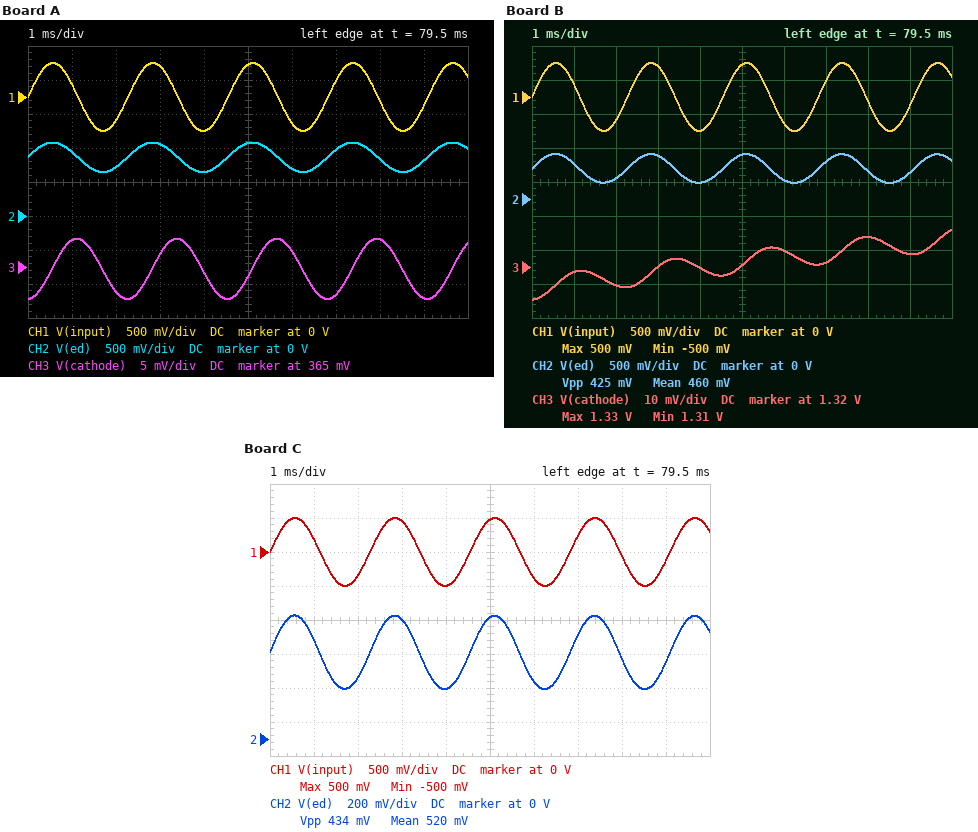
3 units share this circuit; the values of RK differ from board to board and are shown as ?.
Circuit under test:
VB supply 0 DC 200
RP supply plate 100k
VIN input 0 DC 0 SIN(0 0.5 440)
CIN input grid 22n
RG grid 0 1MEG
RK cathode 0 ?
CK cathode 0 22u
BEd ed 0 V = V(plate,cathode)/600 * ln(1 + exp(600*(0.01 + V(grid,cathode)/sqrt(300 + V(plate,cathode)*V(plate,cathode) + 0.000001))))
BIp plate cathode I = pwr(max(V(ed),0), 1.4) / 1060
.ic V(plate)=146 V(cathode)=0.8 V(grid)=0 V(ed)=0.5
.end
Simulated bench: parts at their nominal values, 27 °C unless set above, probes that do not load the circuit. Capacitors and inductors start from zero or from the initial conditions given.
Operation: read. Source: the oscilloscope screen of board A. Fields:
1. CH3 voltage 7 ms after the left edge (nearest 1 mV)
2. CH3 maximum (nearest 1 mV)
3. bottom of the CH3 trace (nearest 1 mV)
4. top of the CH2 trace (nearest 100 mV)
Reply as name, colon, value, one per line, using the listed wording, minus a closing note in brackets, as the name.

CH3 voltage 7 ms after the left edge: 361 mV
CH3 maximum: 369 mV
bottom of the CH3 trace: 360 mV
top of the CH2 trace: 1.1 V
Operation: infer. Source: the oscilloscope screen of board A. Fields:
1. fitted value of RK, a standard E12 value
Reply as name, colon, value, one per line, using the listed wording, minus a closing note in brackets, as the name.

fitted value of RK, a standard E12 value: 470 Ω
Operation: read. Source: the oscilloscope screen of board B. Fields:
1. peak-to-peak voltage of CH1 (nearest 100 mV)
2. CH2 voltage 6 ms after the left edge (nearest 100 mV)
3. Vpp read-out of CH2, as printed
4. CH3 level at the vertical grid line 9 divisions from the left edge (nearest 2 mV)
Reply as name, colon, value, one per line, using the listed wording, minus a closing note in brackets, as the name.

peak-to-peak voltage of CH1: 1.0 V
CH2 voltage 6 ms after the left edge: 300 mV
Vpp read-out of CH2, as printed: 425 mV
CH3 level at the vertical grid line 9 divisions from the left edge: 1.324 V
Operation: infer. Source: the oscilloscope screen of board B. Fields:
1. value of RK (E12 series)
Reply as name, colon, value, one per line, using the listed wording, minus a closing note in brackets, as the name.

value of RK: 4.7 kΩ
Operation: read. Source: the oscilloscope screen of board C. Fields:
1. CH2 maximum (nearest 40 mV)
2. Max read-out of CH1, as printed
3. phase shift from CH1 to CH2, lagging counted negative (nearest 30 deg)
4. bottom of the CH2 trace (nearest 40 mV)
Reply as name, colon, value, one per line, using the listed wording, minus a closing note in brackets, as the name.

CH2 maximum: 720 mV
Max read-out of CH1, as printed: 500 mV
phase shift from CH1 to CH2, lagging counted negative: 0 deg
bottom of the CH2 trace: 280 mV
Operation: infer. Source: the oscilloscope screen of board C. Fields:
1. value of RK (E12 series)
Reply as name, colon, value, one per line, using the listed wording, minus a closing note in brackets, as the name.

value of RK: 3.3 kΩ
